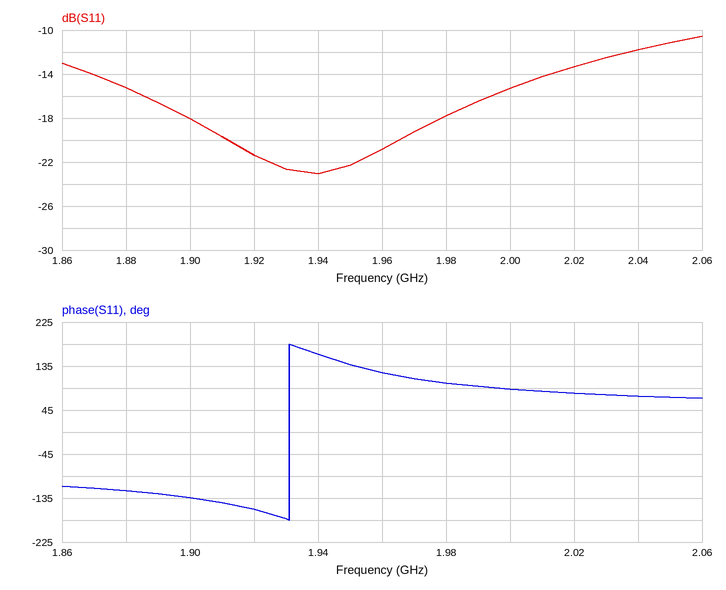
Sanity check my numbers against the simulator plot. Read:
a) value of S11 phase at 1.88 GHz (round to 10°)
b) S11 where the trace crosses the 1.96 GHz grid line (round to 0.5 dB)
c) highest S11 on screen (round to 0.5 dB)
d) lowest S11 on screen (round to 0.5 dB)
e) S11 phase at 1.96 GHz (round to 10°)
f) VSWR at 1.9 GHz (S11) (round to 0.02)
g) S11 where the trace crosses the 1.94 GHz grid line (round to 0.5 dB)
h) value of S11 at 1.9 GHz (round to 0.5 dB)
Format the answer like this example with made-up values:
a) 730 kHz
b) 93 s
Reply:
a) -120°
b) -21.0 dB
c) -10.5 dB
d) -23.0 dB
e) 120°
f) 1.28
g) -23.0 dB
h) -18.0 dB
